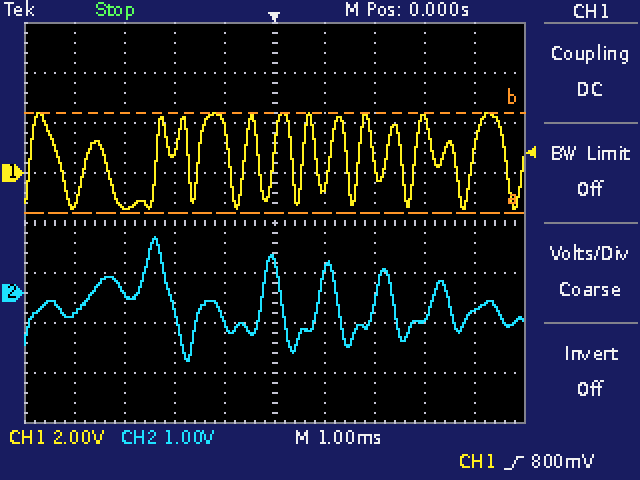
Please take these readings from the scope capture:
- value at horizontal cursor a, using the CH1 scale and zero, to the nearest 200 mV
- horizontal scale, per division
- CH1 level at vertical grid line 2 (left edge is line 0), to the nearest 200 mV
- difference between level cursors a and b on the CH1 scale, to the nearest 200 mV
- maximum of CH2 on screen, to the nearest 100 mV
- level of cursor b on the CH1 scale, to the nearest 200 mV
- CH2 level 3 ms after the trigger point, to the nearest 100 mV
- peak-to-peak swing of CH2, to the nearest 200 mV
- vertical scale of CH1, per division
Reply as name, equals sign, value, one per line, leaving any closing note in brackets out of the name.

value at horizontal cursor a, using the CH1 scale and zero, to the nearest 200 mV = -1.6 V
horizontal scale, per division = 1 ms
CH1 level at vertical grid line 2 (left edge is line 0), to the nearest 200 mV = -1.4 V
difference between level cursors a and b on the CH1 scale, to the nearest 200 mV = 4.0 V
maximum of CH2 on screen, to the nearest 100 mV = 1.1 V
level of cursor b on the CH1 scale, to the nearest 200 mV = 2.4 V
CH2 level 3 ms after the trigger point, to the nearest 100 mV = -500 mV
peak-to-peak swing of CH2, to the nearest 200 mV = 2.4 V
vertical scale of CH1, per division = 2 V
